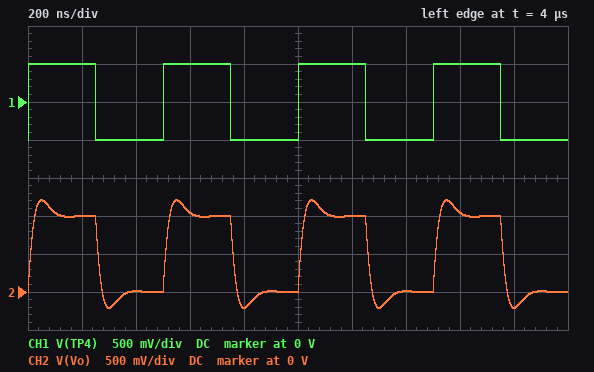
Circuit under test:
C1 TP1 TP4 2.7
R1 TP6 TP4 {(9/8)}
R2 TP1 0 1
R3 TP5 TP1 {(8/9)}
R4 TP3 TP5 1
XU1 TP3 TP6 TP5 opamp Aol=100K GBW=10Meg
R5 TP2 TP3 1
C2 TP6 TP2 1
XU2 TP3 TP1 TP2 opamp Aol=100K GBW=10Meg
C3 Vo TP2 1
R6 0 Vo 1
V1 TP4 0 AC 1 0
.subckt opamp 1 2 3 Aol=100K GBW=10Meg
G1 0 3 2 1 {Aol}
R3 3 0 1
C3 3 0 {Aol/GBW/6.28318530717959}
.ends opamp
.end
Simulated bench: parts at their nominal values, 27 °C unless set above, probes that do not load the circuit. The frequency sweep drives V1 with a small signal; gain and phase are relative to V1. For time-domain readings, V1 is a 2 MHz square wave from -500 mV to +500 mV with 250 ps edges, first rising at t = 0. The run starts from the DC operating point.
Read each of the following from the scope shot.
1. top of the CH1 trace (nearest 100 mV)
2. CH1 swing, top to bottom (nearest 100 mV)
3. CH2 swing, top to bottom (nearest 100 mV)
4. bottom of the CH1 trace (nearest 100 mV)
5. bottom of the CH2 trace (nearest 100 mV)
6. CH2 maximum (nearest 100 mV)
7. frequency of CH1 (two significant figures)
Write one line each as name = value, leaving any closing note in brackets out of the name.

top of the CH1 trace = 500 mV
CH1 swing, top to bottom = 1.0 V
CH2 swing, top to bottom = 1.4 V
bottom of the CH1 trace = -500 mV
bottom of the CH2 trace = -200 mV
CH2 maximum = 1.2 V
frequency of CH1 = 2.0 MHz
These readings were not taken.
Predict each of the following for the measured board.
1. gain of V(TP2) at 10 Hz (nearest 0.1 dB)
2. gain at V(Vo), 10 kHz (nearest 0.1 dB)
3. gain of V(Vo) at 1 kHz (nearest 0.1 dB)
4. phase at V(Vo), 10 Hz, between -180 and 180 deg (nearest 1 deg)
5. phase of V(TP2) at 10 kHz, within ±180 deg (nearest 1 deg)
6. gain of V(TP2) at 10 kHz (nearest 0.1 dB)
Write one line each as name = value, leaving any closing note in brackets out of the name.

gain of V(TP2) at 10 Hz = 0 dB
gain at V(Vo), 10 kHz = 0 dB
gain of V(Vo) at 1 kHz = 0 dB
phase at V(Vo), 10 Hz, between -180 and 180 deg = 1 deg
phase of V(TP2) at 10 kHz, within ±180 deg = 0 deg
gain of V(TP2) at 10 kHz = 0 dB
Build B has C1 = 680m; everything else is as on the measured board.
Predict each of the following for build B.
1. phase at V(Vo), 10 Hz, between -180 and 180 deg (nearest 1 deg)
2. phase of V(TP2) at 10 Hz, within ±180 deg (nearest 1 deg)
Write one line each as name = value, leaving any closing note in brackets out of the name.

phase at V(Vo), 10 Hz, between -180 and 180 deg = 2 deg
phase of V(TP2) at 10 Hz, within ±180 deg = 1 deg
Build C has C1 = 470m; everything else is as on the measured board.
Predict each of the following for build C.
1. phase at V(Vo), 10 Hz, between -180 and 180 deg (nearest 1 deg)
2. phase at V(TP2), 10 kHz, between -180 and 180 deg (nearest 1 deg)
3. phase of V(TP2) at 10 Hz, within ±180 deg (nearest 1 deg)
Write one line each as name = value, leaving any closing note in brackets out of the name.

phase at V(Vo), 10 Hz, between -180 and 180 deg = 3 deg
phase at V(TP2), 10 kHz, between -180 and 180 deg = 0 deg
phase of V(TP2) at 10 Hz, within ±180 deg = 2 deg
